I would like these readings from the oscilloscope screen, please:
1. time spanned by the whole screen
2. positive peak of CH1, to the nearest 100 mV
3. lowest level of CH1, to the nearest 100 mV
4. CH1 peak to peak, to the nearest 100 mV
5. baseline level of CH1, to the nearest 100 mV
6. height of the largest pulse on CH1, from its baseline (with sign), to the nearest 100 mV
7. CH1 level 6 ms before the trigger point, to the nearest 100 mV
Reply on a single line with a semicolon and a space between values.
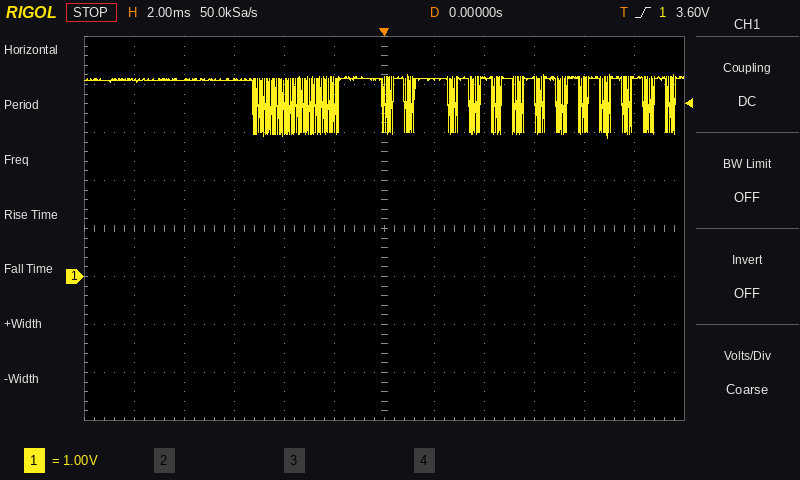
24 ms; 4.2 V; 2.9 V; 1.3 V; 4.1 V; -1.2 V; 4.1 V
